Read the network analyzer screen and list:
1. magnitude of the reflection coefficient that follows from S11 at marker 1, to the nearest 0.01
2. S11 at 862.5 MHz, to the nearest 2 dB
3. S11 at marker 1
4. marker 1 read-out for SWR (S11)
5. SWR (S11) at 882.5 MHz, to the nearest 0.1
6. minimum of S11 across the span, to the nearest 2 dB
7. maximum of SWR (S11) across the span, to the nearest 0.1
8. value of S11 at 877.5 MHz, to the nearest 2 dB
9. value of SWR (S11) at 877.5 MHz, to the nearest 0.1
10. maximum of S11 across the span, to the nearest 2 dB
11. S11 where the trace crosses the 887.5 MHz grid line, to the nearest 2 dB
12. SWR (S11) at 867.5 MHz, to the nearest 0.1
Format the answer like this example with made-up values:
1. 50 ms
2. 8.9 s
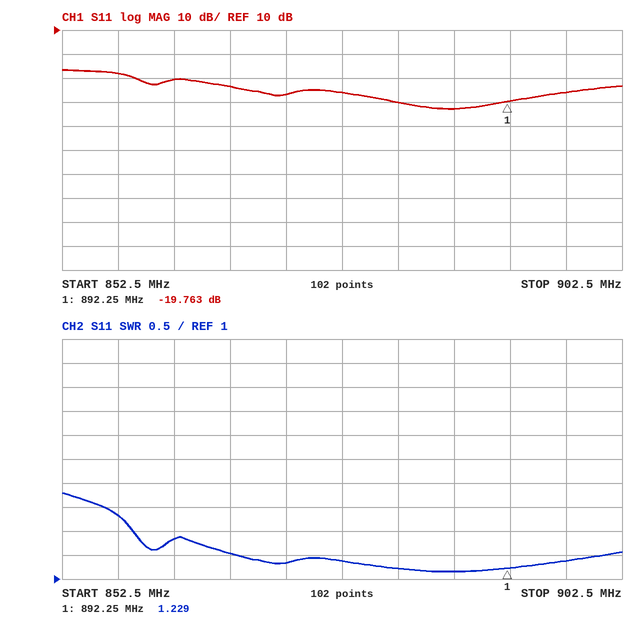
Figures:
1. 0.10
2. -10 dB
3. -19.763 dB
4. 1.229
5. 1.2
6. -22 dB
7. 2.8
8. -16 dB
9. 1.4
10. -6 dB
11. -22 dB
12. 1.5
